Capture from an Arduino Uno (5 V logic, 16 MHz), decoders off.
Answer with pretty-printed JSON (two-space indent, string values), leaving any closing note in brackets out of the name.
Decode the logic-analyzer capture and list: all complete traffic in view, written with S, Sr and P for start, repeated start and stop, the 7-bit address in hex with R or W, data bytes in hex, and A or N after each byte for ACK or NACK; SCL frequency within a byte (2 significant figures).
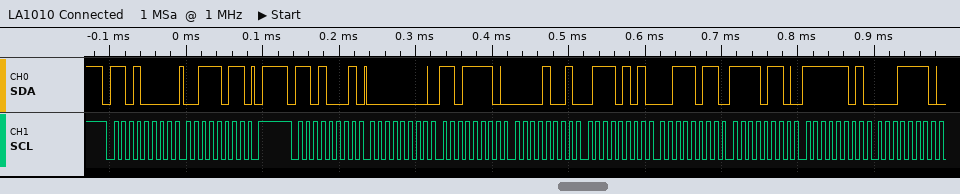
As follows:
{
  "all complete traffic in view, written with S, Sr and P for start, repeated start and stop, the 7-bit address in hex with R or W, data bytes in hex, and A or N after each byte for ACK or NACK": "S 68W A 3B A P S 68R A 00 A DE A 09 A 75 A 3B A F6 A FD A 1E A",
  "SCL frequency within a byte": "100 kHz"
}
